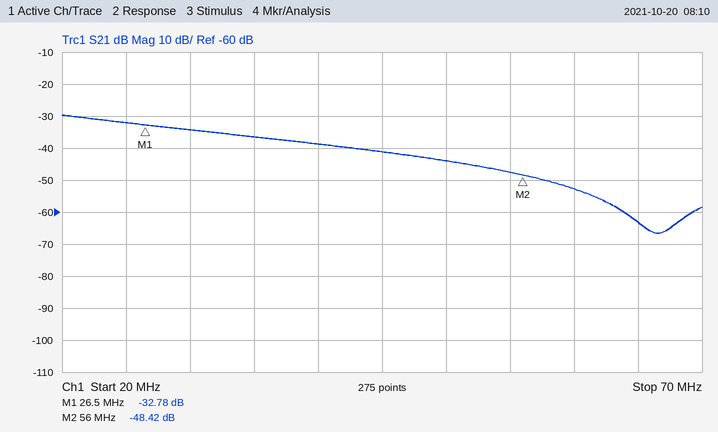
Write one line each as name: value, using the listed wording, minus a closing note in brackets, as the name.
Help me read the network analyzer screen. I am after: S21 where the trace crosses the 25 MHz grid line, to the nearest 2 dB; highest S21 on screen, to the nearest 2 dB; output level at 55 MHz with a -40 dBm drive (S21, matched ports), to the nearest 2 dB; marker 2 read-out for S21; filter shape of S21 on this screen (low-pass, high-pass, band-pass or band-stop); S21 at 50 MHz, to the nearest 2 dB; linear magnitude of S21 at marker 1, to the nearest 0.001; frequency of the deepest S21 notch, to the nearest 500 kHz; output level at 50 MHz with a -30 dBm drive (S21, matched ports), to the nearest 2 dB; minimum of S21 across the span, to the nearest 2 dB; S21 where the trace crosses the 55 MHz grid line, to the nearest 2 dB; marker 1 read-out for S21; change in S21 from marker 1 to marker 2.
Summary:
S21 where the trace crosses the 25 MHz grid line, to the nearest 2 dB: -32 dB
highest S21 on screen, to the nearest 2 dB: -30 dB
output level at 55 MHz with a -40 dBm drive (S21, matched ports), to the nearest 2 dB: -88 dBm
marker 2 read-out for S21: -48.42 dB
filter shape of S21 on this screen: low-pass
S21 at 50 MHz, to the nearest 2 dB: -44 dB
linear magnitude of S21 at marker 1, to the nearest 0.001: 0.023
frequency of the deepest S21 notch, to the nearest 500 kHz: 66.5 MHz
output level at 50 MHz with a -30 dBm drive (S21, matched ports), to the nearest 2 dB: -74 dBm
minimum of S21 across the span, to the nearest 2 dB: -66 dB
S21 where the trace crosses the 55 MHz grid line, to the nearest 2 dB: -48 dB
marker 1 read-out for S21: -32.78 dB
change in S21 from marker 1 to marker 2: -15.64 dB
